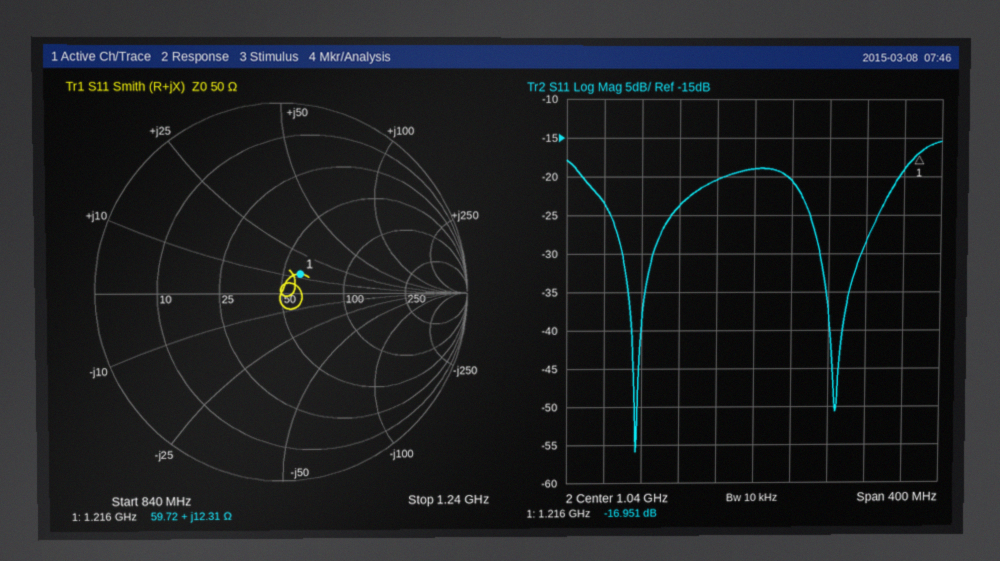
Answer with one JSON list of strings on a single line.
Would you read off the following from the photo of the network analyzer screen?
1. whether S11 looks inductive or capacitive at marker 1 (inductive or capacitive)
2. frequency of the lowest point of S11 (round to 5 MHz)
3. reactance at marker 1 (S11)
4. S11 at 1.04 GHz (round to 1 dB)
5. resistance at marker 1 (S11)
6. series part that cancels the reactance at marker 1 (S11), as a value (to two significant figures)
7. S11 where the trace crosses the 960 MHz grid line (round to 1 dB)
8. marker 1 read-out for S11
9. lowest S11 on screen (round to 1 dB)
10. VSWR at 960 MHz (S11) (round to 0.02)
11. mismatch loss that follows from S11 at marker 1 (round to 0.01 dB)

["inductive", "915 MHz", "+12.31 Ω", "-19 dB", "59.72 Ω", "11 pF", "-24 dB", "-16.951 dB", "-56 dB", "1.14", "0.09 dB"]
